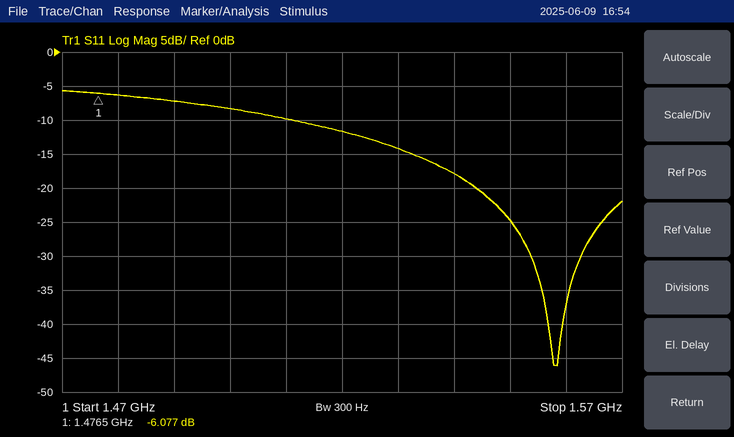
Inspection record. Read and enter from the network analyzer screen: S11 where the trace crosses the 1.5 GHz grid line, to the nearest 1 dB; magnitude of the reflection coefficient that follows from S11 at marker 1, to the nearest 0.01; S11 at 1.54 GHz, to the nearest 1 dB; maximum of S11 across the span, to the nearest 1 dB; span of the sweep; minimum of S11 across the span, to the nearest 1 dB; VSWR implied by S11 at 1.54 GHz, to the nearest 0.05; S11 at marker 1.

-8 dB
0.50
-18 dB
-6 dB
100 MHz
-46 dB
1.30
-6.077 dB
